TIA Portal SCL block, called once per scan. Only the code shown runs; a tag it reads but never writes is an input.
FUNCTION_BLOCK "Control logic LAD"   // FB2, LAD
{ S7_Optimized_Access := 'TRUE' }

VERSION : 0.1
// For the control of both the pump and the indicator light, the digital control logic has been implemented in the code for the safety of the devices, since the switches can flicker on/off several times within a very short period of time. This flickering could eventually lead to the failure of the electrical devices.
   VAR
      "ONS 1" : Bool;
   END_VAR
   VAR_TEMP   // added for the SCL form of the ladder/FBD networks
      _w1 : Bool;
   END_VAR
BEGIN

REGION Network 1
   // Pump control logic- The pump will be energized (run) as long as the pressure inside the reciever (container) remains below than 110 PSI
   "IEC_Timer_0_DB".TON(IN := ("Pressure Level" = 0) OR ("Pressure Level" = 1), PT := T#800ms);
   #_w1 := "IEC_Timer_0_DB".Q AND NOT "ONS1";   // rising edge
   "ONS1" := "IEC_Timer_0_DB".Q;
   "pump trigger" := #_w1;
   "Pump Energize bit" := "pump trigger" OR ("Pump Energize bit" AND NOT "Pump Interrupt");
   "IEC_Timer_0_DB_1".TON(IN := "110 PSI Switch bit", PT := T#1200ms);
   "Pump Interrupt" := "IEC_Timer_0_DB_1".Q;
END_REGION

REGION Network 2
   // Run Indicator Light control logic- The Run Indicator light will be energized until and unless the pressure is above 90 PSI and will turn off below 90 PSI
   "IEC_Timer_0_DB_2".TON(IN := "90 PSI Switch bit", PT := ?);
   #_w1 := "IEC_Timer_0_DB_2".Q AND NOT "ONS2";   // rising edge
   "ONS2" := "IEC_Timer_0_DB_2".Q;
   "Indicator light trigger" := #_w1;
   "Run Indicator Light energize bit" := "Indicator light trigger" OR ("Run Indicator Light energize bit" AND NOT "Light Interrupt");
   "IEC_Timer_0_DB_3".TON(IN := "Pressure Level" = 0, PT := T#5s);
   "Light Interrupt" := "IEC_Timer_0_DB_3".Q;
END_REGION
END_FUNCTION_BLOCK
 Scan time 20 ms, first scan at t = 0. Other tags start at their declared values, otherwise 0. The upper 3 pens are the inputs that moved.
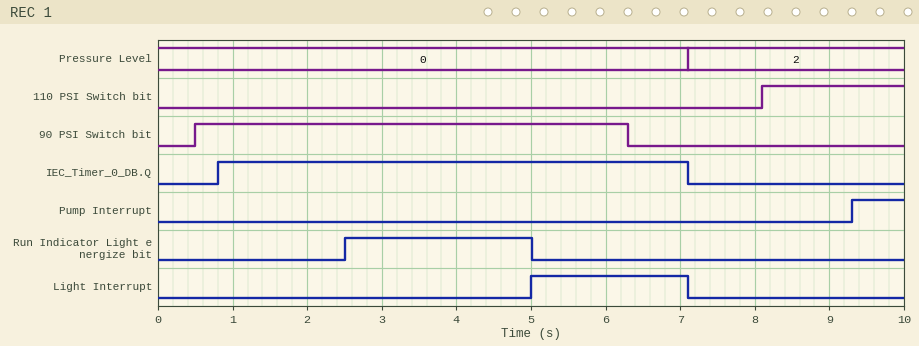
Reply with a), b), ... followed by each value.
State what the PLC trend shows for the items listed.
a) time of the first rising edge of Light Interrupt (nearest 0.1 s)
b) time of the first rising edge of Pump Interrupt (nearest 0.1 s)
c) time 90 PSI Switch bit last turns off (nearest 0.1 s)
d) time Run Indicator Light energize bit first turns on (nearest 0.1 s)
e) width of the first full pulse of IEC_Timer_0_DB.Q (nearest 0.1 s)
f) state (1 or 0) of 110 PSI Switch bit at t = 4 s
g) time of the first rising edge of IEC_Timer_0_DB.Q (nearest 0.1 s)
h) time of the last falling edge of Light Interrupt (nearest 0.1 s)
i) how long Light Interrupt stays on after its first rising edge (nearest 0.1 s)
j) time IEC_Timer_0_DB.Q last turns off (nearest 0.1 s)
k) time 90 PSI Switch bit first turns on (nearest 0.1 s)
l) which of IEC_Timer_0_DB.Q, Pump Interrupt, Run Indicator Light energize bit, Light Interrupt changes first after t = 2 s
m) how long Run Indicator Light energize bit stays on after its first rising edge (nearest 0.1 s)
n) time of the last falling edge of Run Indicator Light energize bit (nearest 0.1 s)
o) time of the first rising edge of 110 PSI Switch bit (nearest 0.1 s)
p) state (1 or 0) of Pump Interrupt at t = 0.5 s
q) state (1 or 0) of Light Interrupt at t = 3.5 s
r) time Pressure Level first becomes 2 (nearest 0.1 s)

a) 5.0 s
b) 9.3 s
c) 6.3 s
d) 2.5 s
e) 6.3 s
f) 0
g) 0.8 s
h) 7.1 s
i) 2.1 s
j) 7.1 s
k) 0.5 s
l) Run Indicator Light energize bit
m) 2.5 s
n) 5.0 s
o) 8.1 s
p) 0
q) 0
r) 7.1 s
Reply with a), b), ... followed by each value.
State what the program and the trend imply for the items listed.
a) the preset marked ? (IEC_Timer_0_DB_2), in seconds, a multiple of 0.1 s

a) 2.0 s
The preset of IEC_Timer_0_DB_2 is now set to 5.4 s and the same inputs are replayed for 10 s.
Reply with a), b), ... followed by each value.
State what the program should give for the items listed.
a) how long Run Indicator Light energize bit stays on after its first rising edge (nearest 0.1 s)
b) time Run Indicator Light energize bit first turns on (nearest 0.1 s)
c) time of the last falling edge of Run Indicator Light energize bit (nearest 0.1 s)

a) 0.0 s
b) 5.9 s
c) 5.9 s
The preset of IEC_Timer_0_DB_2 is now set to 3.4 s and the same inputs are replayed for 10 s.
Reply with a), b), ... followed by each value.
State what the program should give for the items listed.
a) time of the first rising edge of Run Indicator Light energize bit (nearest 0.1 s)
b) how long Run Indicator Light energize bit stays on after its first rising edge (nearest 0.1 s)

a) 3.9 s
b) 1.1 s
